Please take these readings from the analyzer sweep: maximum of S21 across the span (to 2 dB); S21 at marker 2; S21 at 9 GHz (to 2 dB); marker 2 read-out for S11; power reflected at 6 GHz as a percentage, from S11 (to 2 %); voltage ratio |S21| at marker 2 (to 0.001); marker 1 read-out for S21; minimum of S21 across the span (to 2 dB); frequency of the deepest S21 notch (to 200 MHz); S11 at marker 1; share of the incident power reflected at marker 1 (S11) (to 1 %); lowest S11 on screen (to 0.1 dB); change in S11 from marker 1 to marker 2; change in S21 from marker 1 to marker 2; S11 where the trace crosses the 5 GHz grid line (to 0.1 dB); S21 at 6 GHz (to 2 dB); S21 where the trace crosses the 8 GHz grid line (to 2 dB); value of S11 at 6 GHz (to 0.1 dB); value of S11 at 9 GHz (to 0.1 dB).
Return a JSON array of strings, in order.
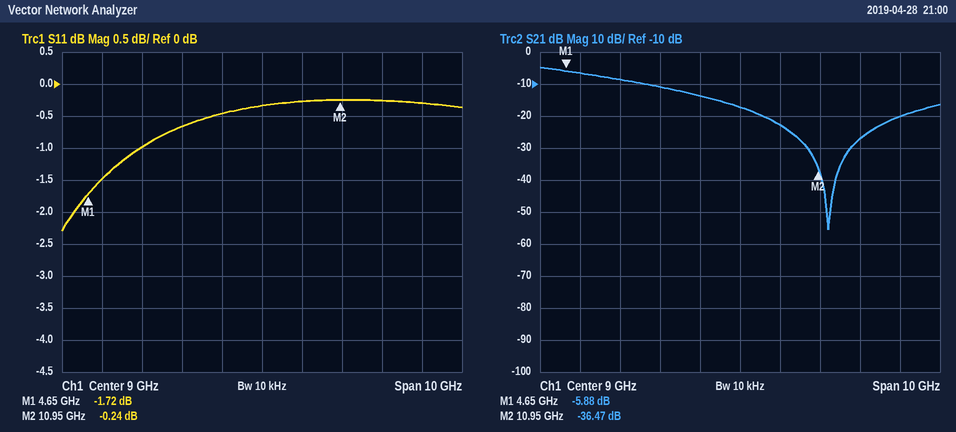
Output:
["-4 dB", "-36.47 dB", "-18 dB", "-0.24 dB", "80 %", "0.015", "-5.88 dB", "-56 dB", "11.2 GHz", "-1.72 dB", "67 %", "-2.3 dB", "1.48 dB", "-30.59 dB", "-1.5 dB", "-8 dB", "-14 dB", "-1.0 dB", "-0.3 dB"]
